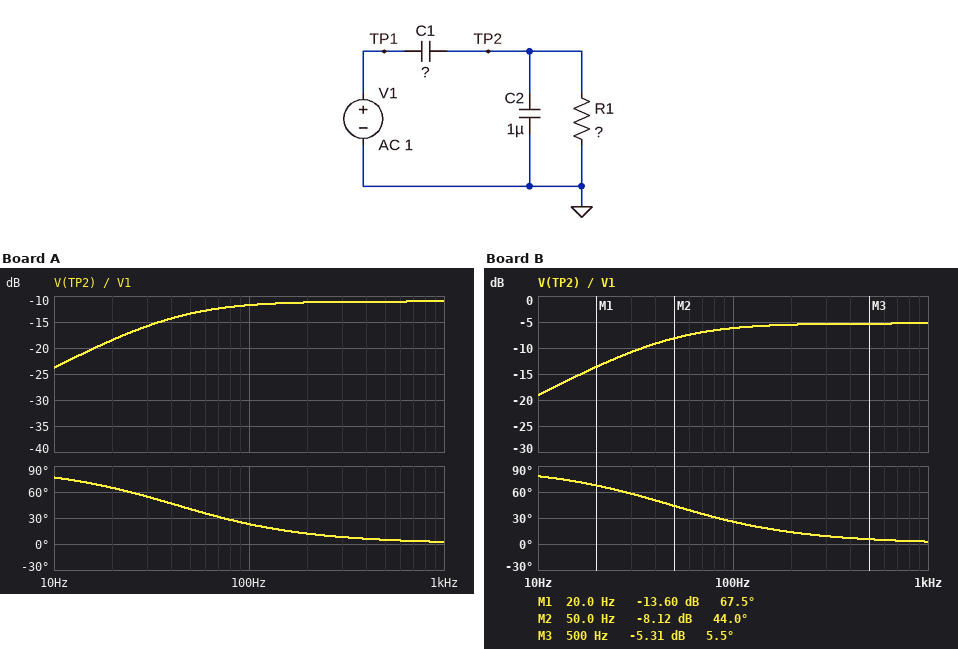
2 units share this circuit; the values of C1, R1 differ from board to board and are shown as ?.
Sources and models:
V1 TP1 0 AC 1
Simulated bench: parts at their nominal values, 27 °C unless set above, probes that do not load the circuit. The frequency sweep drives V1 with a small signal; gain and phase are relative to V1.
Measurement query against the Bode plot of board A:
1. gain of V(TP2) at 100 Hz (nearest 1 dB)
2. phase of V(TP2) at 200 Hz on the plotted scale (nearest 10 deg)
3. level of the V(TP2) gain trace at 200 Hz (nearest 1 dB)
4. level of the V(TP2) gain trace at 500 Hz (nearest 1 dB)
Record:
-12 dB
10 deg
-11 dB
-11 dB
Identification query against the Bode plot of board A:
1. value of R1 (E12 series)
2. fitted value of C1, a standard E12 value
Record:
2.7 kΩ
390 nF
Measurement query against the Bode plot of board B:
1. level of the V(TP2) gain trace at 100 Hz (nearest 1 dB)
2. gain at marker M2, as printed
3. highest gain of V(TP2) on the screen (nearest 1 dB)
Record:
-6 dB
-8.12 dB
-5 dB
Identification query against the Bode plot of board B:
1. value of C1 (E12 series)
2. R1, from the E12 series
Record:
1.2 µF
1.5 kΩ
